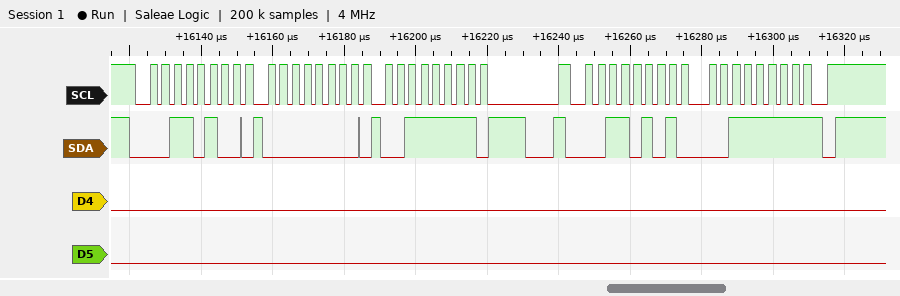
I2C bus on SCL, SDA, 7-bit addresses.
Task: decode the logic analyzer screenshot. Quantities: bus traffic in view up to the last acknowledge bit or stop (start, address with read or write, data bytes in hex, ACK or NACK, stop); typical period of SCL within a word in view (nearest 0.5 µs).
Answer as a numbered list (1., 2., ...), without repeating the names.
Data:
1. start, address 1A write ACK, 00 ACK, 3F ACK, repeated start, address 1A read ACK, 3F NACK, stop
2. 3.5 µs
